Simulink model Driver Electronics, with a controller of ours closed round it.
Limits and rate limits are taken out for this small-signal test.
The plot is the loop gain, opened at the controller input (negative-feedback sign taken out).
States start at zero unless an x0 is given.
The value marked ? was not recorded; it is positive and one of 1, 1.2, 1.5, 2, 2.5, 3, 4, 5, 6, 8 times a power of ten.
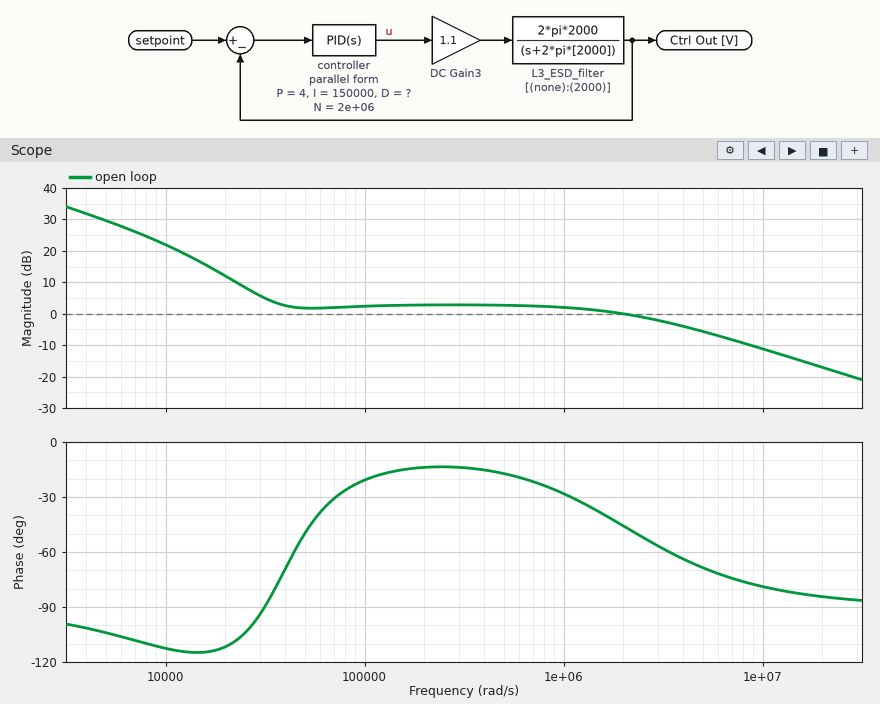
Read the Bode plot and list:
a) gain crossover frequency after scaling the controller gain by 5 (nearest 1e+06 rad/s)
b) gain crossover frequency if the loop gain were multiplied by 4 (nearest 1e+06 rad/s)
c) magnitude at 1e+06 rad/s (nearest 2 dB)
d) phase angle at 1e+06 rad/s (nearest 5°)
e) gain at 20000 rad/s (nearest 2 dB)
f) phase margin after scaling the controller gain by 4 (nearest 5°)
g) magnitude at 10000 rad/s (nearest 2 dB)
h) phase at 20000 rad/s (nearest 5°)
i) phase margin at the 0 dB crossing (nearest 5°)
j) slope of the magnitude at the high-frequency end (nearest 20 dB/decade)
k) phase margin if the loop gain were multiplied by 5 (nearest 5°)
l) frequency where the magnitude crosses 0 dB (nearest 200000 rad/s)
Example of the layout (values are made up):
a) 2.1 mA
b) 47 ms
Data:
a) 14000000 rad/s
b) 11000000 rad/s
c) 2 dB
d) -30°
e) 12 dB
f) 100°
g) 22 dB
h) -110°
i) 135°
j) -20 dB/decade
k) 100°
l) 2000000 rad/s
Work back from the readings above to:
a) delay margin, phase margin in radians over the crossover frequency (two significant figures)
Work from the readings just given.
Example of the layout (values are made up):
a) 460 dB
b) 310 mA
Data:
a) 0.0000012 s
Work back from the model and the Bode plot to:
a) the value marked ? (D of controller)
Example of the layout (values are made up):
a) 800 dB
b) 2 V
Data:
a) 0.0001
